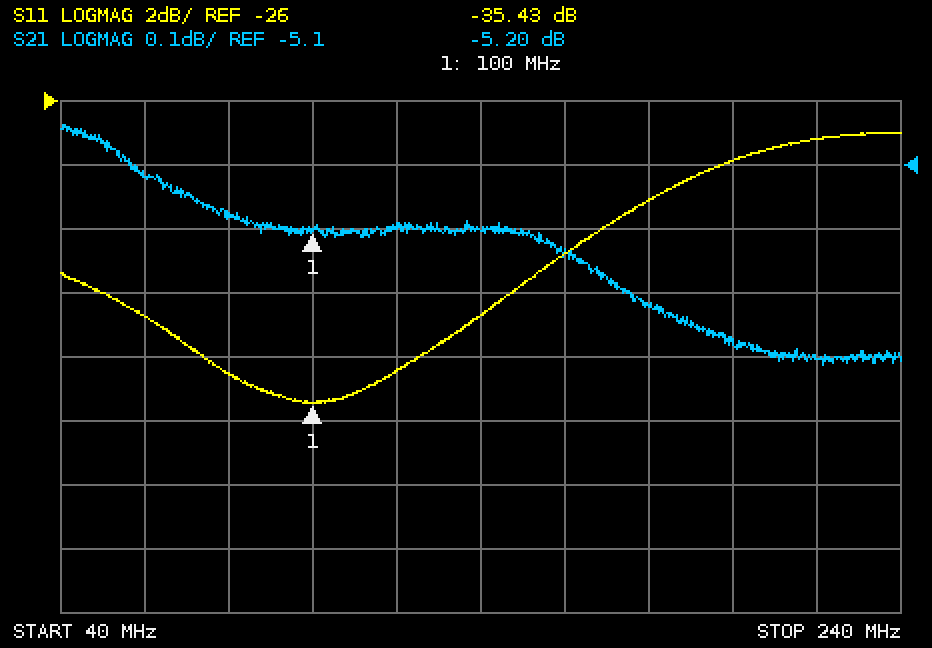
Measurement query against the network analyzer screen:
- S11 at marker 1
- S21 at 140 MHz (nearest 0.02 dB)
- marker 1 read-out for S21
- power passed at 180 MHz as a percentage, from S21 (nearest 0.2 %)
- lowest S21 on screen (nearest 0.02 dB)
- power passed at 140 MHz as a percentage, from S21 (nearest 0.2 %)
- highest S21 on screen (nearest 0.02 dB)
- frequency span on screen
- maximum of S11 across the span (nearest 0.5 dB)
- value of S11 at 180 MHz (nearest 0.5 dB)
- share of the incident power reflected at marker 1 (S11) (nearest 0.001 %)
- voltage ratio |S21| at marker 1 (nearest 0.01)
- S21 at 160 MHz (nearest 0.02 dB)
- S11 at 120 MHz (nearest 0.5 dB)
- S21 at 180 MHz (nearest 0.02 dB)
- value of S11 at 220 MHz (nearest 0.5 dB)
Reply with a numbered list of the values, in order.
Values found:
1. -35.43 dB
2. -5.20 dB
3. -5.20 dB
4. 29.4 %
5. -5.42 dB
6. 30.2 %
7. -5.04 dB
8. 200 MHz
9. -27.0 dB
10. -29.0 dB
11. 0.029 %
12. 0.55
13. -5.24 dB
14. -34.5 dB
15. -5.32 dB
16. -27.0 dB
